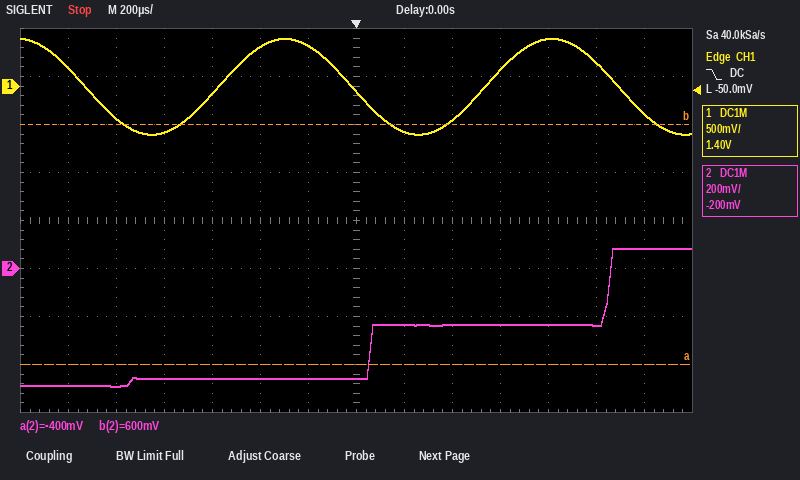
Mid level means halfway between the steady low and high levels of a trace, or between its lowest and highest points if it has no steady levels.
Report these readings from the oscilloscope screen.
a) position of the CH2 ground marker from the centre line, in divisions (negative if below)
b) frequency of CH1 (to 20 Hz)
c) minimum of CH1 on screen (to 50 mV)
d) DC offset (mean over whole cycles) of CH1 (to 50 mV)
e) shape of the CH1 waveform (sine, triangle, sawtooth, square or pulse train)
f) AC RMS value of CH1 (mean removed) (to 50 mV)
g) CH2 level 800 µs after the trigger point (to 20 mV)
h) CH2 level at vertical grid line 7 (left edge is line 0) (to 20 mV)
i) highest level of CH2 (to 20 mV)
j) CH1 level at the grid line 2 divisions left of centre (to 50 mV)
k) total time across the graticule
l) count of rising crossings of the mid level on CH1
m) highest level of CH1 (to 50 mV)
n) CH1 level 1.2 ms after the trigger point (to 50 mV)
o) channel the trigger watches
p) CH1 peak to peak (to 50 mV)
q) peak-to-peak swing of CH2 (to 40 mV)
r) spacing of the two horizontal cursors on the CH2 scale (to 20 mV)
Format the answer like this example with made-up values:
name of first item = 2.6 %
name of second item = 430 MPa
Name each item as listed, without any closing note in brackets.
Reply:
position of the CH2 ground marker from the centre line, in divisions = -1.0 div
frequency of CH1 = 900 Hz
minimum of CH1 on screen = -500 mV
DC offset (mean over whole cycles) of CH1 = 0 mV
shape of the CH1 waveform = sine
AC RMS value of CH1 (mean removed) = 350 mV
CH2 level 800 µs after the trigger point = -240 mV
CH2 level at vertical grid line 7 (left edge is line 0) = -460 mV
highest level of CH2 = 80 mV
CH1 level at the grid line 2 divisions left of centre = 400 mV
total time across the graticule = 2.8 ms
count of rising crossings of the mid level on CH1 = 2
highest level of CH1 = 500 mV
CH1 level 1.2 ms after the trigger point = -300 mV
channel the trigger watches = CH1
CH1 peak to peak = 1.00 V
peak-to-peak swing of CH2 = 560 mV
spacing of the two horizontal cursors on the CH2 scale = 1.00 V
